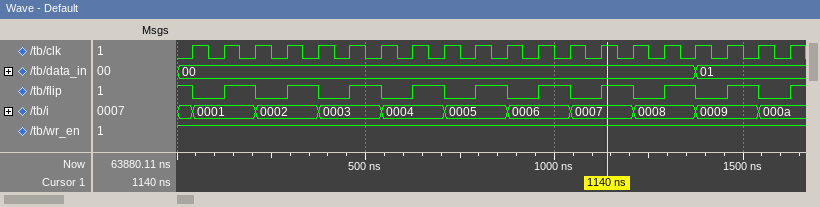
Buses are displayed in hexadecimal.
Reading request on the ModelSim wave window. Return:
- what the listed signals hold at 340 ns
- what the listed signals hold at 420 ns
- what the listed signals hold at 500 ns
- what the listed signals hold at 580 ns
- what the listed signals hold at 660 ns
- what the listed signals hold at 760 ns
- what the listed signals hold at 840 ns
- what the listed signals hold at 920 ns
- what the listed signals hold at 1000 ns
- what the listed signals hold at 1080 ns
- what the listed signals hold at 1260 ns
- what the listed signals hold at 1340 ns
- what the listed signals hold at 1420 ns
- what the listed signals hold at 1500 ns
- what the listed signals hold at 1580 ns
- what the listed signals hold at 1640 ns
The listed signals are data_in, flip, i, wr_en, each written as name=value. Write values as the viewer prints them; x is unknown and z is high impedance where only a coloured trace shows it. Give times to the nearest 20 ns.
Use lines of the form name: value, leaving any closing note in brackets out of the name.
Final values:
what the listed signals hold at 340 ns: data_in=00, flip=1, i=0002, wr_en=1
what the listed signals hold at 420 ns: data_in=00, flip=0, i=0003, wr_en=1
what the listed signals hold at 500 ns: data_in=00, flip=1, i=0003, wr_en=1
what the listed signals hold at 580 ns: data_in=00, flip=0, i=0004, wr_en=1
what the listed signals hold at 660 ns: data_in=00, flip=1, i=0004, wr_en=1
what the listed signals hold at 760 ns: data_in=00, flip=0, i=0005, wr_en=1
what the listed signals hold at 840 ns: data_in=00, flip=1, i=0005, wr_en=1
what the listed signals hold at 920 ns: data_in=00, flip=0, i=0006, wr_en=1
what the listed signals hold at 1000 ns: data_in=00, flip=1, i=0006, wr_en=1
what the listed signals hold at 1080 ns: data_in=00, flip=0, i=0007, wr_en=1
what the listed signals hold at 1260 ns: data_in=00, flip=0, i=0008, wr_en=1
what the listed signals hold at 1340 ns: data_in=00, flip=1, i=0008, wr_en=1
what the listed signals hold at 1420 ns: data_in=01, flip=0, i=0009, wr_en=1
what the listed signals hold at 1500 ns: data_in=01, flip=1, i=0009, wr_en=1
what the listed signals hold at 1580 ns: data_in=01, flip=0, i=000a, wr_en=1
what the listed signals hold at 1640 ns: data_in=01, flip=1, i=000a, wr_en=1
